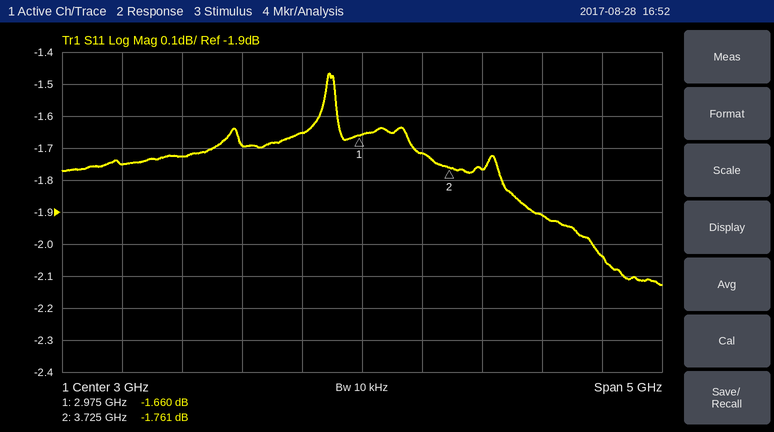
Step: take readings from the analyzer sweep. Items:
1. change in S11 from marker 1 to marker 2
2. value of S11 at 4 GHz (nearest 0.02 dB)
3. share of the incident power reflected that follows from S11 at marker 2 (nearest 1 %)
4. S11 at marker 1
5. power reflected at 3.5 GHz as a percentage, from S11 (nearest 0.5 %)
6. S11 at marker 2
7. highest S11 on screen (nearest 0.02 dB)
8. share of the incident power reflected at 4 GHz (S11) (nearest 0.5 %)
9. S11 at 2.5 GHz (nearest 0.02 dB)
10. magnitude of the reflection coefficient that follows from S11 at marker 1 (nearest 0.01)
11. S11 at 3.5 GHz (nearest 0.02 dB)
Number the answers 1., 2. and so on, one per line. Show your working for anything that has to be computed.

1. -1.761 − (-1.66) = -0.101 dB
2. -1.76 dB
3. 10^(-1.761/10) ≈ 67 %
4. -1.660 dB
5. 10^(-1.72/10) ≈ 67.3 %, so 67.5 % to the nearest 0.5 %
6. -1.761 dB
7. -1.46 dB
8. 10^(-1.76/10) ≈ 66.7 %, so 66.5 % to the nearest 0.5 %
9. -1.66 dB
10. 10^(-1.66/20) ≈ 0.83
11. -1.72 dB
